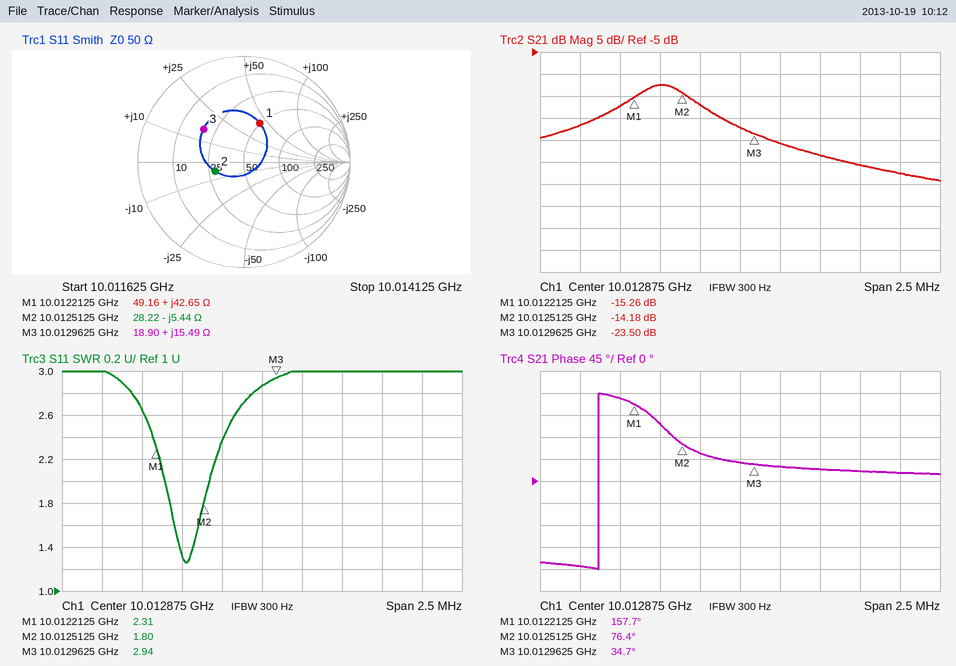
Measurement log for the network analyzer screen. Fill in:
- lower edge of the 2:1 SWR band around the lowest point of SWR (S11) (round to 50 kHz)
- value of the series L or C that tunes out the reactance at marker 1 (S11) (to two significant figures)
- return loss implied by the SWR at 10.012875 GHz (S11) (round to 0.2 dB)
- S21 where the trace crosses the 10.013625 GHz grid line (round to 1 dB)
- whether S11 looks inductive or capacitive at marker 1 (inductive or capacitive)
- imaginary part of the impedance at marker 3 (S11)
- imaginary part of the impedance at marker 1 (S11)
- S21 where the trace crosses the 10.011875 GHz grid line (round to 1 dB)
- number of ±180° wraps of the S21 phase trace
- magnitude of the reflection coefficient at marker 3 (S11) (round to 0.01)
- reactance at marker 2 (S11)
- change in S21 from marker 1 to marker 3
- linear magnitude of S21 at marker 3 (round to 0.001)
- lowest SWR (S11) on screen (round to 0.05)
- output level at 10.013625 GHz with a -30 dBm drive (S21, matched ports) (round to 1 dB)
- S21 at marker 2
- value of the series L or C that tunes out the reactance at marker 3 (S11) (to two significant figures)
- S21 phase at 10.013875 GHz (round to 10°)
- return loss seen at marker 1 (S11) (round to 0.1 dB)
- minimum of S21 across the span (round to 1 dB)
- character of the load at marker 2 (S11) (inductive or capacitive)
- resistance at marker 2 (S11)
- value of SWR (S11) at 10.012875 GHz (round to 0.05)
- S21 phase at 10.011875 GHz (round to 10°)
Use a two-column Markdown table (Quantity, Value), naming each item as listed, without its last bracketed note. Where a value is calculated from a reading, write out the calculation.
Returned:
| Quantity | Value |
|---|---|
| lower edge of the 2:1 SWR band around the lowest point of SWR (S11) | 10.01225 GHz |
| value of the series L or C that tunes out the reactance at marker 1 (S11) | C = 1/(2π × 10.0122125 GHz × 42.65 Ω) ≈ 373 fF, so 370 fF to two significant figures |
| return loss implied by the SWR at 10.012875 GHz (S11) | −20 log10((2.85 − 1)/(2.85 + 1)) ≈ 6.4 dB |
| S21 where the trace crosses the 10.013625 GHz grid line | -31 dB |
| whether S11 looks inductive or capacitive at marker 1 | inductive |
| imaginary part of the impedance at marker 3 | +15.49 Ω |
| imaginary part of the impedance at marker 1 | +42.65 Ω |
| S21 where the trace crosses the 10.011875 GHz grid line | -22 dB |
| number of ±180° wraps of the S21 phase trace | 1 |
| magnitude of the reflection coefficient at marker 3 (S11) | 0.49 |
| reactance at marker 2 | -5.44 Ω |
| change in S21 from marker 1 to marker 3 | -23.5 − (-15.26) = -8.24 dB |
| linear magnitude of S21 at marker 3 | 10^(-23.5/20) ≈ 0.067 |
| lowest SWR (S11) on screen | 1.25 |
| output level at 10.013625 GHz with a -30 dBm drive (S21, matched ports) | -30 dBm + (-31 dB) = -61 dBm |
| S21 at marker 2 | -14.18 dB |
| value of the series L or C that tunes out the reactance at marker 3 (S11) | C = 1/(2π × 10.0129625 GHz × 15.49 Ω) ≈ 1.0 pF |
| S21 phase at 10.013875 GHz | 20° |
| return loss seen at marker 1 (S11) | 8.1 dB |
| minimum of S21 across the span | -34 dB |
| character of the load at marker 2 (S11) | capacitive |
| resistance at marker 2 | 28.22 Ω |
| value of SWR (S11) at 10.012875 GHz | 2.85 |
| S21 phase at 10.011875 GHz | -170° |
